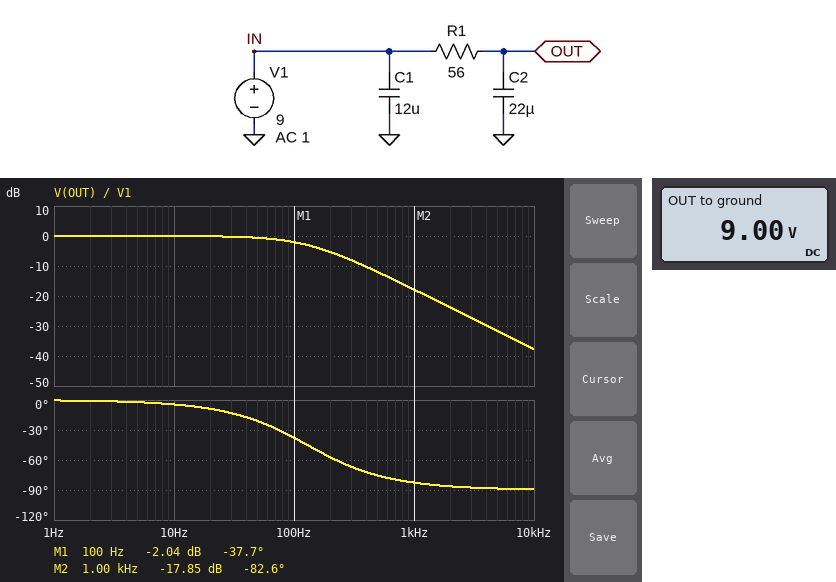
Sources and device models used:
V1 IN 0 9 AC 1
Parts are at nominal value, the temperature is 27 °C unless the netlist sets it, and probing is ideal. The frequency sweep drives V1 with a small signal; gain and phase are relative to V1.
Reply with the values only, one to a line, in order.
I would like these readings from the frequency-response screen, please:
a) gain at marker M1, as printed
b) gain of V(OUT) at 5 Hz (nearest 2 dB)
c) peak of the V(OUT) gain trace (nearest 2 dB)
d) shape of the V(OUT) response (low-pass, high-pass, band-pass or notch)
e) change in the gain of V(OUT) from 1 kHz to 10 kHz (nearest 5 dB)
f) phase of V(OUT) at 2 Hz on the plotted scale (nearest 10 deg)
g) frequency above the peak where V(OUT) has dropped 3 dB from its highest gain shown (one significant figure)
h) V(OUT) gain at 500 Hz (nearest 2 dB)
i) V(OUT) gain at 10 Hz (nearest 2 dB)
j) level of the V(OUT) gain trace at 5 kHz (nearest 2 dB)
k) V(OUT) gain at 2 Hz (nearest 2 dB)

-2.04 dB
0 dB
0 dB
low-pass
-20 dB
0 deg
100 Hz
-12 dB
0 dB
-32 dB
0 dB
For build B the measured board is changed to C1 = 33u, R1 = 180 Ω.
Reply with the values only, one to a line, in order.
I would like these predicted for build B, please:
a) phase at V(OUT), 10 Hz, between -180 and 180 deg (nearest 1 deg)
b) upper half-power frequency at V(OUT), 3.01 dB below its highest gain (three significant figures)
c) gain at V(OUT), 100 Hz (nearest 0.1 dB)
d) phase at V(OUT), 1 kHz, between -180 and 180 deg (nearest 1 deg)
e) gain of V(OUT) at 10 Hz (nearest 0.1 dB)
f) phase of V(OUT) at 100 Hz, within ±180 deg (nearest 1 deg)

-14 deg
40.2 Hz
-8.6 dB
-88 deg
-0.3 dB
-68 deg
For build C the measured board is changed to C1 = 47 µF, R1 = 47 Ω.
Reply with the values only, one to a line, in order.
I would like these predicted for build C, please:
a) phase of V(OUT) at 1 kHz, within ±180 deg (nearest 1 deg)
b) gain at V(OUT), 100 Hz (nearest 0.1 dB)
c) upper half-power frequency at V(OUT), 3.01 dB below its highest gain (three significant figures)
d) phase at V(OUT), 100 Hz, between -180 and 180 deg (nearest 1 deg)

-81 deg
-1.5 dB
154 Hz
-33 deg
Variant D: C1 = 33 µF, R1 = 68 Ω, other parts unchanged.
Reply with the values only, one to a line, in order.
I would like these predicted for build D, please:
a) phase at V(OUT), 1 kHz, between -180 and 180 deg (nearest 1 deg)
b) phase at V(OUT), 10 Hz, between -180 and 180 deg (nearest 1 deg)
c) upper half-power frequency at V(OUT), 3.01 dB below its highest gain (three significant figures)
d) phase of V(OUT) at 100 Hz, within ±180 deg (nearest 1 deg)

-84 deg
-5 deg
106 Hz
-43 deg
